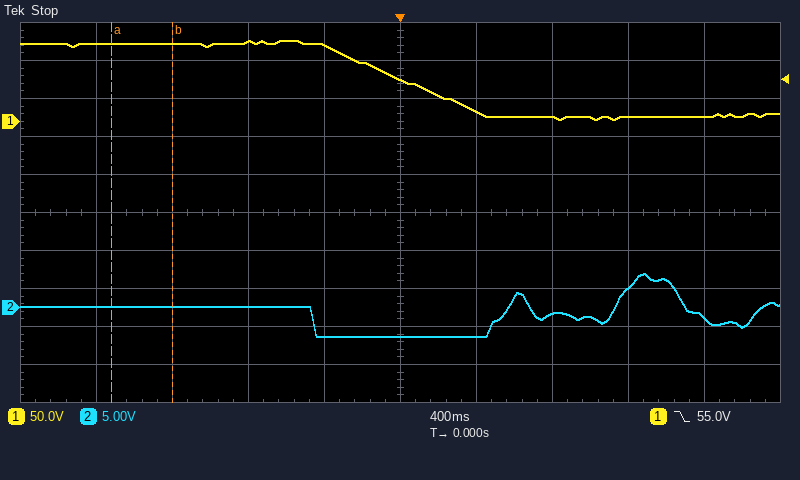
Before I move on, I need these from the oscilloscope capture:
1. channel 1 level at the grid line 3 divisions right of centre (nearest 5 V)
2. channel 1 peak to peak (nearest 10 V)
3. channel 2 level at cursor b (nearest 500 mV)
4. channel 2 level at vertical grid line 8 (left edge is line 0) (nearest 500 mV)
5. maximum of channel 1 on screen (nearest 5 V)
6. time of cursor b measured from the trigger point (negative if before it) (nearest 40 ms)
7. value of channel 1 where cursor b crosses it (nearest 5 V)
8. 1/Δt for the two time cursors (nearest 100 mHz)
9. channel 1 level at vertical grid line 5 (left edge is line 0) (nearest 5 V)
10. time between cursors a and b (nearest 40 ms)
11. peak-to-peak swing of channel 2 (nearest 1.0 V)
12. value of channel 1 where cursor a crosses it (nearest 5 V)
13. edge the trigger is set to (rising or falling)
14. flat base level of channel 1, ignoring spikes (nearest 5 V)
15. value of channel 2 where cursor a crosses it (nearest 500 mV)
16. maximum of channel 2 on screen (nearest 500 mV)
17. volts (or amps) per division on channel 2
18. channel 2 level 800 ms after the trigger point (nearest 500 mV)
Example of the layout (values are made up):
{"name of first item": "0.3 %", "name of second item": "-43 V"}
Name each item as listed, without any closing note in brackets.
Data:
{"channel 1 level at the grid line 3 divisions right of centre": "5 V", "channel 1 peak to peak": "100 V", "channel 2 level at cursor b": "0.0 V", "channel 2 level at vertical grid line 8 (left edge is line 0)": "2.5 V", "maximum of channel 1 on screen": "105 V", "time of cursor b measured from the trigger point (negative if before it)": "-1.20 s", "value of channel 1 where cursor b crosses it": "100 V", "1/Δt for the two time cursors": "3.1 Hz", "channel 1 level at vertical grid line 5 (left edge is line 0)": "55 V", "time between cursors a and b": "320 ms", "peak-to-peak swing of channel 2": "8.0 V", "value of channel 1 where cursor a crosses it": "100 V", "edge the trigger is set to": "falling", "flat base level of channel 1, ignoring spikes": "5 V", "value of channel 2 where cursor a crosses it": "0.0 V", "maximum of channel 2 on screen": "4.5 V", "volts (or amps) per division on channel 2": "5 V", "channel 2 level 800 ms after the trigger point": "-1.0 V"}
